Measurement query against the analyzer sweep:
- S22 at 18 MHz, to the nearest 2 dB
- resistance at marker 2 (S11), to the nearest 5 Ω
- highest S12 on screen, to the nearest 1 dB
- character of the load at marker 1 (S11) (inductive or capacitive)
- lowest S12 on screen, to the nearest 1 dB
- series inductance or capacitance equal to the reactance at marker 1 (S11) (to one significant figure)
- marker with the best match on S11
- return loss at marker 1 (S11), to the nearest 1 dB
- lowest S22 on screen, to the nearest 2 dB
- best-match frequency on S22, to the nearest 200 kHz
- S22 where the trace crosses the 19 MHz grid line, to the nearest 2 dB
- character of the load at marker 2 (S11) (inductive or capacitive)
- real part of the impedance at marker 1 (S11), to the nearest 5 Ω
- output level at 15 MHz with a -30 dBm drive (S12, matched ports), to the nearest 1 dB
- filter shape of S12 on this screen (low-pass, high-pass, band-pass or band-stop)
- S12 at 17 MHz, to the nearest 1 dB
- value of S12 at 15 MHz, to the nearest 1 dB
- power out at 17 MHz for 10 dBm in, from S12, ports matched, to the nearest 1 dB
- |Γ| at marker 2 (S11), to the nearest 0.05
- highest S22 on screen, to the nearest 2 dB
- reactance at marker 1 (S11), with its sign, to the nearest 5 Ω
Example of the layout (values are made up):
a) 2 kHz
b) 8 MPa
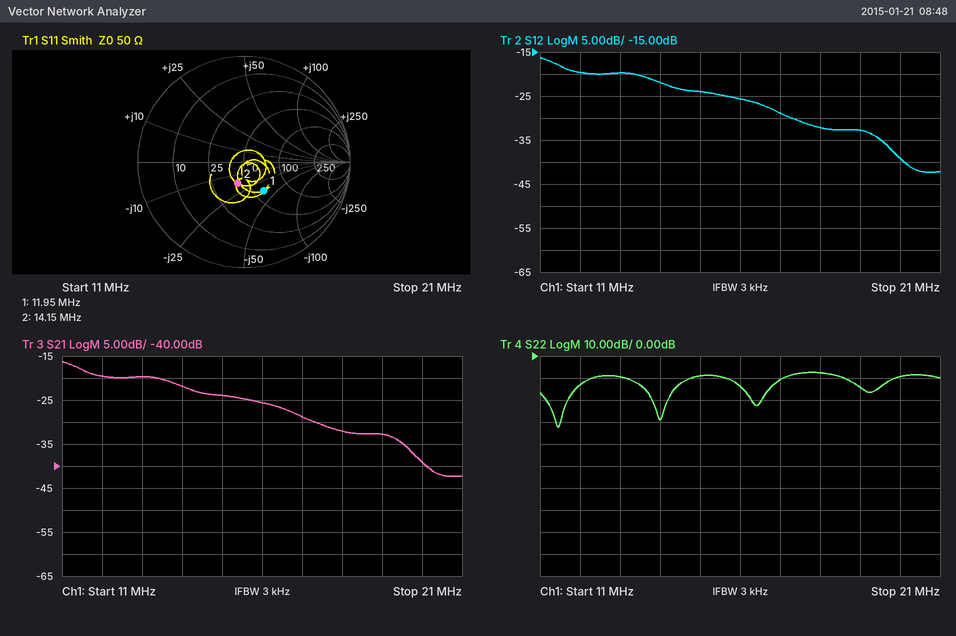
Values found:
a) -8 dB
b) 40 Ω
c) -16 dB
d) capacitive
e) -42 dB
f) 400 pF
g) marker 2
h) 10 dB
i) -32 dB
j) 11.4 MHz
k) -14 dB
l) capacitive
m) 60 Ω
n) -54 dBm
o) low-pass
p) -29 dB
q) -24 dB
r) -19 dBm
s) 0.20
t) -8 dB
u) -35 Ω
